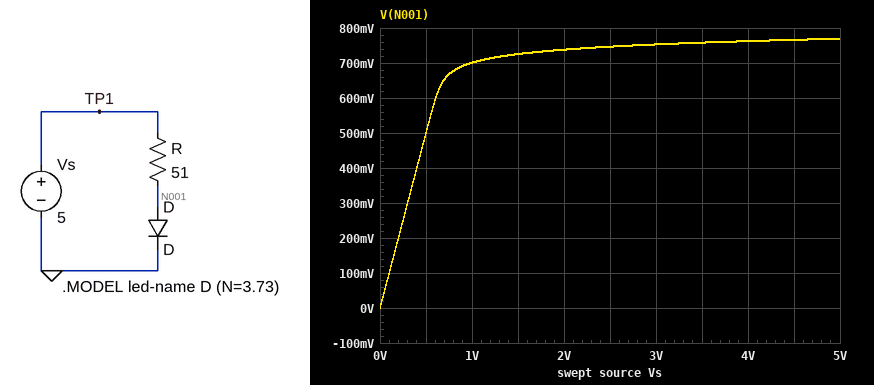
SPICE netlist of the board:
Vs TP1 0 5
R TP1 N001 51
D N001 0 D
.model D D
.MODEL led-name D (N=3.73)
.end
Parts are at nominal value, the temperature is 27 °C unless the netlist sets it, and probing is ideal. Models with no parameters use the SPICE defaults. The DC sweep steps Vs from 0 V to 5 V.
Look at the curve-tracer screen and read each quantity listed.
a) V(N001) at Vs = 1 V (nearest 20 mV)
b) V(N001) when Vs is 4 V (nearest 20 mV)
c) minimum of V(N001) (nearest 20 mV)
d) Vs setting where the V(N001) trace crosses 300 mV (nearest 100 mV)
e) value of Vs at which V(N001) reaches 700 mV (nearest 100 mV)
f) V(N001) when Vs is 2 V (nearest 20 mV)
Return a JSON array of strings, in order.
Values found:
["700 mV", "760 mV", "0 V", "300 mV", "1.0 V", "740 mV"]
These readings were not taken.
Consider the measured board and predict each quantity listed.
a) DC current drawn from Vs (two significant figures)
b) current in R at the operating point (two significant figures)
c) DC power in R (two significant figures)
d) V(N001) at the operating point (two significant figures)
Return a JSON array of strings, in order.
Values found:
["83 mA", "83 mA", "350 mW", "770 mV"]
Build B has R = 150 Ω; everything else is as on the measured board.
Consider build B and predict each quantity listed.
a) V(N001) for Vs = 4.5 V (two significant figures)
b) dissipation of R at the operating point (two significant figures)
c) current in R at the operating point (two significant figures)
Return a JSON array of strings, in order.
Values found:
["740 mV", "120 mW", "28 mA"]
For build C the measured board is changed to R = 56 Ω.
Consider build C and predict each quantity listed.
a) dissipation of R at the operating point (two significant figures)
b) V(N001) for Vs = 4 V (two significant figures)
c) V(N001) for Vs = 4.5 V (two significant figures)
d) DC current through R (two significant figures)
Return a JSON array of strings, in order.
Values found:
["320 mW", "760 mV", "760 mV", "76 mA"]
